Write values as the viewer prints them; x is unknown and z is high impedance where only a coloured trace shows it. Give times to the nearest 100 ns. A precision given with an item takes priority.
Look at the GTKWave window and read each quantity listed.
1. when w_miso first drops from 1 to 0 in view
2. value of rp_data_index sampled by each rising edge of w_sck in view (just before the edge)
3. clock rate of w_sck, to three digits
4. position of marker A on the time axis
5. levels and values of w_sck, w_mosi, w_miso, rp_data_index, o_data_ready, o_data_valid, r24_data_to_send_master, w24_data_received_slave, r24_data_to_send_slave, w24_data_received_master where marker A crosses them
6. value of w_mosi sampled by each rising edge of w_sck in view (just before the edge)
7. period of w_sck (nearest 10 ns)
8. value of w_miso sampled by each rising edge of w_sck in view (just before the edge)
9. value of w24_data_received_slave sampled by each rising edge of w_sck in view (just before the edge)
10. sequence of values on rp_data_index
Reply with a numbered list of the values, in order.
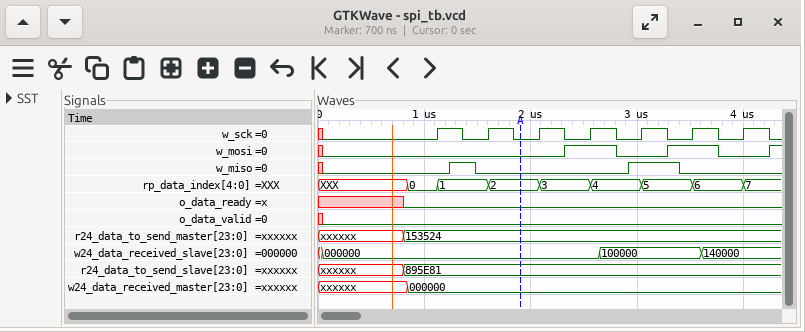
1. 1500 ns
2. 0, 1, 2, 3, 4, 5, 6
3. 2.08 MHz
4. 1900 ns
5. w_sck=0, w_mosi=0, w_miso=0, rp_data_index=2, o_data_ready=0, o_data_valid=0, r24_data_to_send_master=153524, w24_data_received_slave=000000, r24_data_to_send_slave=895E81, w24_data_received_master=000000
6. 0 0 0 1 0 1 0
7. 480 ns
8. 0 0 0 0 1 0 0
9. 000000, 000000, 000000, 000000, 100000, 100000, 140000
10. XXX, 0, 1, 2, 3, 4, 5, 6, 7
